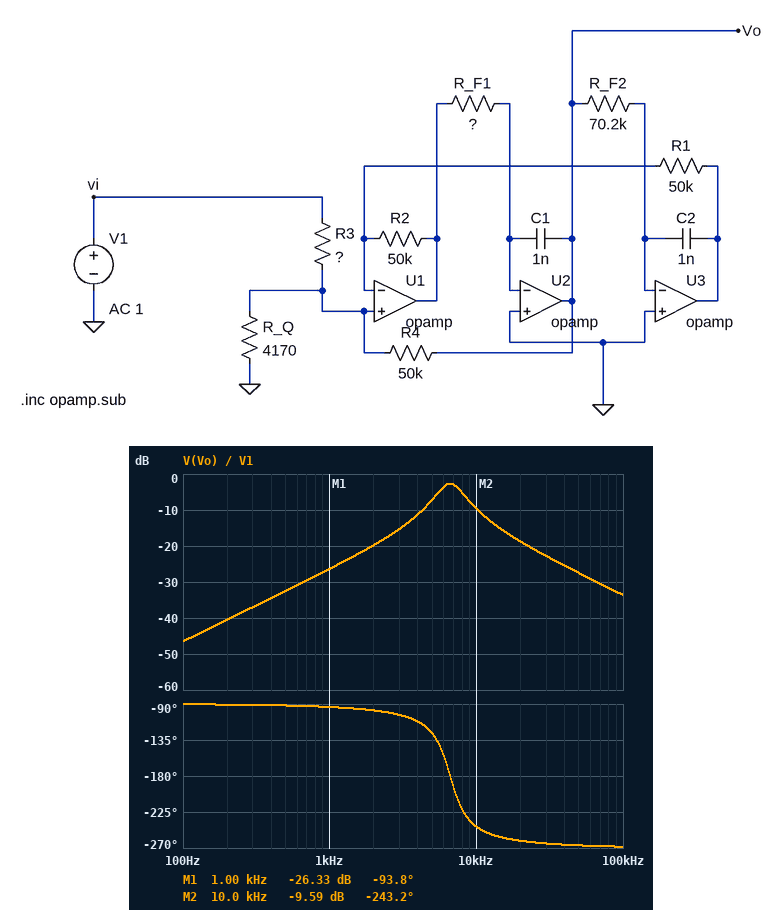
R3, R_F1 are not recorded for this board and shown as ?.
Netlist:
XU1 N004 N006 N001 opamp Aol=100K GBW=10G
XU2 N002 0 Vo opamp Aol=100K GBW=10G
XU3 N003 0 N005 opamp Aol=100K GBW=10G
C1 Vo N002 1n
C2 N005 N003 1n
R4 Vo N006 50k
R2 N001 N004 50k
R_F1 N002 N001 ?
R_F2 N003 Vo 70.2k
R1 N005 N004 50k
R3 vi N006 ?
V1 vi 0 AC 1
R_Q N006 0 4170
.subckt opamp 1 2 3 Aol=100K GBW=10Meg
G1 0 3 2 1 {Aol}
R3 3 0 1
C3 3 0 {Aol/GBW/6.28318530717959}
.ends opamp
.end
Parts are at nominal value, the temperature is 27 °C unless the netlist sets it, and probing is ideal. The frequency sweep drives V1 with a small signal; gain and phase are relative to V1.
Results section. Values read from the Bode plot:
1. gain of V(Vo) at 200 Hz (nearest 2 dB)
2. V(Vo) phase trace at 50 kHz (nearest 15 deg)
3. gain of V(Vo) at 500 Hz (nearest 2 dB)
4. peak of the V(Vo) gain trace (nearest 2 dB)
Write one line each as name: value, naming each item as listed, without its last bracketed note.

gain of V(Vo) at 200 Hz: -40 dB
V(Vo) phase trace at 50 kHz: -270 deg
gain of V(Vo) at 500 Hz: -32 dB
peak of the V(Vo) gain trace: -2 dB
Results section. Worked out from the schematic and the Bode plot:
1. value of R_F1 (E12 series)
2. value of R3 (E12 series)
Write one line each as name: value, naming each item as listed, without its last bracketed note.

value of R_F1: 8.2 kΩ
value of R3: 68 kΩ
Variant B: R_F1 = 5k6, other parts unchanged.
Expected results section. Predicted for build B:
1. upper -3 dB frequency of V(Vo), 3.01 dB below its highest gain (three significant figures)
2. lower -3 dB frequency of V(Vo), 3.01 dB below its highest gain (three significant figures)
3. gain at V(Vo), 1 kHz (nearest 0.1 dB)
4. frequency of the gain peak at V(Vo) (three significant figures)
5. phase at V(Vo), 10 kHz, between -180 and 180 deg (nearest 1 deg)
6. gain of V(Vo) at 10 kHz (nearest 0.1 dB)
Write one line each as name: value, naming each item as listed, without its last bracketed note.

upper -3 dB frequency of V(Vo), 3.01 dB below its highest gain: 10.4 kHz
lower -3 dB frequency of V(Vo), 3.01 dB below its highest gain: 6.22 kHz
gain at V(Vo), 1 kHz: -26.4 dB
frequency of the gain peak at V(Vo): 8.03 kHz
phase at V(Vo), 10 kHz, between -180 and 180 deg: 139 deg
gain of V(Vo) at 10 kHz: -5.1 dB
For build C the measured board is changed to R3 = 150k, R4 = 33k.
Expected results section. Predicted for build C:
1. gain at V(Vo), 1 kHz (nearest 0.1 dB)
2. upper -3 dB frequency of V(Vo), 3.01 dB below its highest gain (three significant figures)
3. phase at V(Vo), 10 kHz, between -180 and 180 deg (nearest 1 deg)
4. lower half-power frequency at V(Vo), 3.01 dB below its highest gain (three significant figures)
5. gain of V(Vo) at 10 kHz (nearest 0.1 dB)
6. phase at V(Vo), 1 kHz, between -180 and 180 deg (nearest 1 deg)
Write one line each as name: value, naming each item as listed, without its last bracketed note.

gain at V(Vo), 1 kHz: -33.3 dB
upper -3 dB frequency of V(Vo), 3.01 dB below its highest gain: 9.09 kHz
phase at V(Vo), 10 kHz, between -180 and 180 deg: 127 deg
lower half-power frequency at V(Vo), 3.01 dB below its highest gain: 4.84 kHz
gain of V(Vo) at 10 kHz: -17.5 dB
phase at V(Vo), 1 kHz, between -180 and 180 deg: -96 deg
